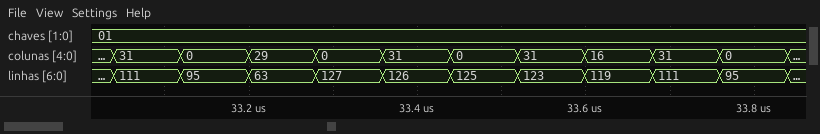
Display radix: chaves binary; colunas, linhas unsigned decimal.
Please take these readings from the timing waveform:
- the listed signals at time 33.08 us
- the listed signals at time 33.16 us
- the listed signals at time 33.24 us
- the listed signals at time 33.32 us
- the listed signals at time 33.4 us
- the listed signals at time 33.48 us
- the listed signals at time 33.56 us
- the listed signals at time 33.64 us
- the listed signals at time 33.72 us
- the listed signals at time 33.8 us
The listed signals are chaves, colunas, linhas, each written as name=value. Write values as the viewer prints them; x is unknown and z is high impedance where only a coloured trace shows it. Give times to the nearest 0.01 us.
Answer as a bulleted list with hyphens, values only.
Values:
- chaves=01, colunas=31, linhas=111
- chaves=01, colunas=0, linhas=95
- chaves=01, colunas=29, linhas=63
- chaves=01, colunas=0, linhas=127
- chaves=01, colunas=31, linhas=126
- chaves=01, colunas=0, linhas=125
- chaves=01, colunas=31, linhas=123
- chaves=01, colunas=16, linhas=119
- chaves=01, colunas=31, linhas=111
- chaves=01, colunas=0, linhas=95
